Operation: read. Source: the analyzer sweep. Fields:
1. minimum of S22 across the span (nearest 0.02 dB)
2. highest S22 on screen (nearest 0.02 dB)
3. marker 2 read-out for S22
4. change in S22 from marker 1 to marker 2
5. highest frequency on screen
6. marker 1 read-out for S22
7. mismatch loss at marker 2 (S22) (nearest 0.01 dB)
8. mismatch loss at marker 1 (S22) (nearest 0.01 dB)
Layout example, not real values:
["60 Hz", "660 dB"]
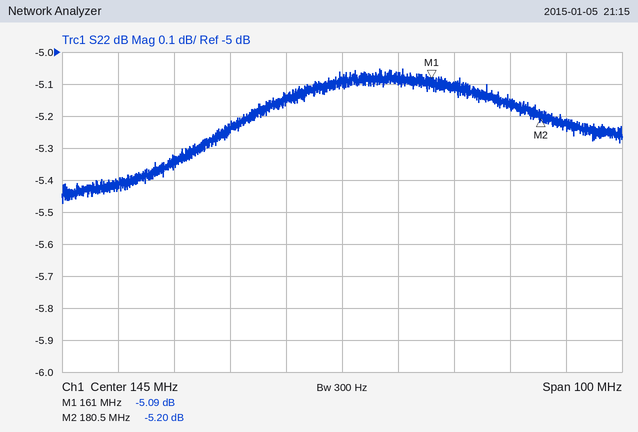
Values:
["-5.48 dB", "-5.06 dB", "-5.20 dB", "-0.11 dB", "195 MHz", "-5.09 dB", "1.56 dB", "1.61 dB"]
